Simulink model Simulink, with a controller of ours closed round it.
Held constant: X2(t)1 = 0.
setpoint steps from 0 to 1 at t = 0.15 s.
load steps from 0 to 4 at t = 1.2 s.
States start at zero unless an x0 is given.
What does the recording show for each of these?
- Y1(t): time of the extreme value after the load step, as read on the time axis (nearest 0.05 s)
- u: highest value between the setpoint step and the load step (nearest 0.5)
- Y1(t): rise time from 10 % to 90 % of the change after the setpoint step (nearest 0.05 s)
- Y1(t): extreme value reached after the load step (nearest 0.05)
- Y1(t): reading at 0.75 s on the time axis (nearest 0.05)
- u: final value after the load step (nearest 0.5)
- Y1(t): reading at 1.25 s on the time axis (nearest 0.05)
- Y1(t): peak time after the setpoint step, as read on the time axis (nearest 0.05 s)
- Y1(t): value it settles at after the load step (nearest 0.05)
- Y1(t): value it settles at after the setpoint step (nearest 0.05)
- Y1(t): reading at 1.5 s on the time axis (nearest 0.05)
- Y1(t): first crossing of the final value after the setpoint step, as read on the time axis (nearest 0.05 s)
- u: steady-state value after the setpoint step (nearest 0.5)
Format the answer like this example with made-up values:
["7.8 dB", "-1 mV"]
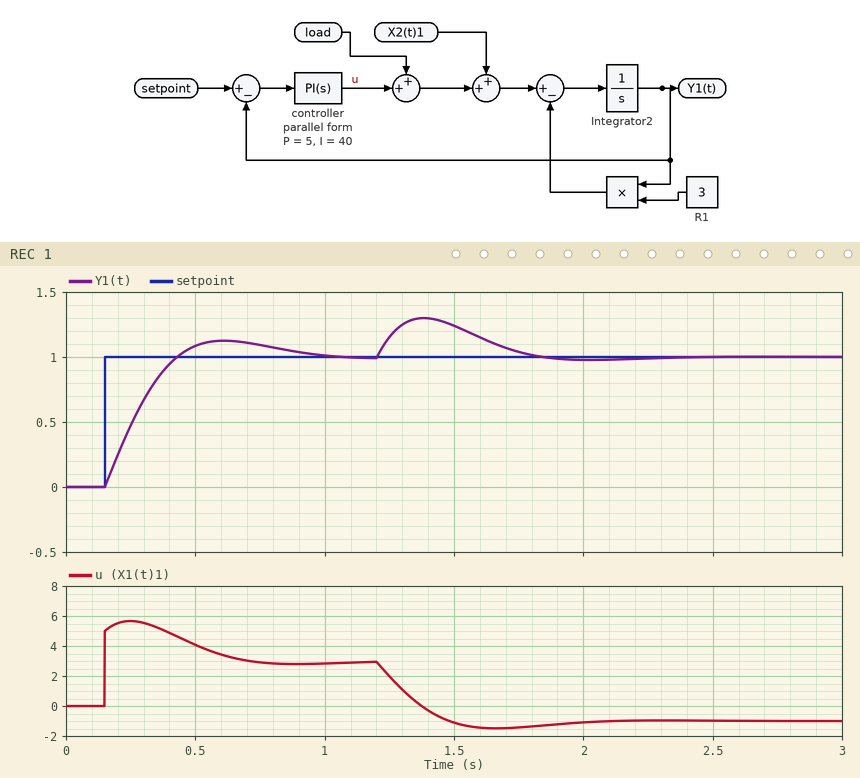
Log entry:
["1.40 s", "5.5", "0.20 s", "1.30", "1.10", "-1.0", "1.15", "0.60 s", "1.00", "1.00", "1.25", "0.45 s", "3.0"]
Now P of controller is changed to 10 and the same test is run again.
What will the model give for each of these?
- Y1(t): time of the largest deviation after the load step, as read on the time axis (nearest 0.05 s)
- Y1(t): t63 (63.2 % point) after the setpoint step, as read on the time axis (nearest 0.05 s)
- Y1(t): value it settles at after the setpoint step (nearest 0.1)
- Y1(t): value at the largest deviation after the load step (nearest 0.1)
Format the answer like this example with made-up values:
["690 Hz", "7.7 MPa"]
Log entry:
["1.35 s", "0.25 s", "1.0", "1.2"]
